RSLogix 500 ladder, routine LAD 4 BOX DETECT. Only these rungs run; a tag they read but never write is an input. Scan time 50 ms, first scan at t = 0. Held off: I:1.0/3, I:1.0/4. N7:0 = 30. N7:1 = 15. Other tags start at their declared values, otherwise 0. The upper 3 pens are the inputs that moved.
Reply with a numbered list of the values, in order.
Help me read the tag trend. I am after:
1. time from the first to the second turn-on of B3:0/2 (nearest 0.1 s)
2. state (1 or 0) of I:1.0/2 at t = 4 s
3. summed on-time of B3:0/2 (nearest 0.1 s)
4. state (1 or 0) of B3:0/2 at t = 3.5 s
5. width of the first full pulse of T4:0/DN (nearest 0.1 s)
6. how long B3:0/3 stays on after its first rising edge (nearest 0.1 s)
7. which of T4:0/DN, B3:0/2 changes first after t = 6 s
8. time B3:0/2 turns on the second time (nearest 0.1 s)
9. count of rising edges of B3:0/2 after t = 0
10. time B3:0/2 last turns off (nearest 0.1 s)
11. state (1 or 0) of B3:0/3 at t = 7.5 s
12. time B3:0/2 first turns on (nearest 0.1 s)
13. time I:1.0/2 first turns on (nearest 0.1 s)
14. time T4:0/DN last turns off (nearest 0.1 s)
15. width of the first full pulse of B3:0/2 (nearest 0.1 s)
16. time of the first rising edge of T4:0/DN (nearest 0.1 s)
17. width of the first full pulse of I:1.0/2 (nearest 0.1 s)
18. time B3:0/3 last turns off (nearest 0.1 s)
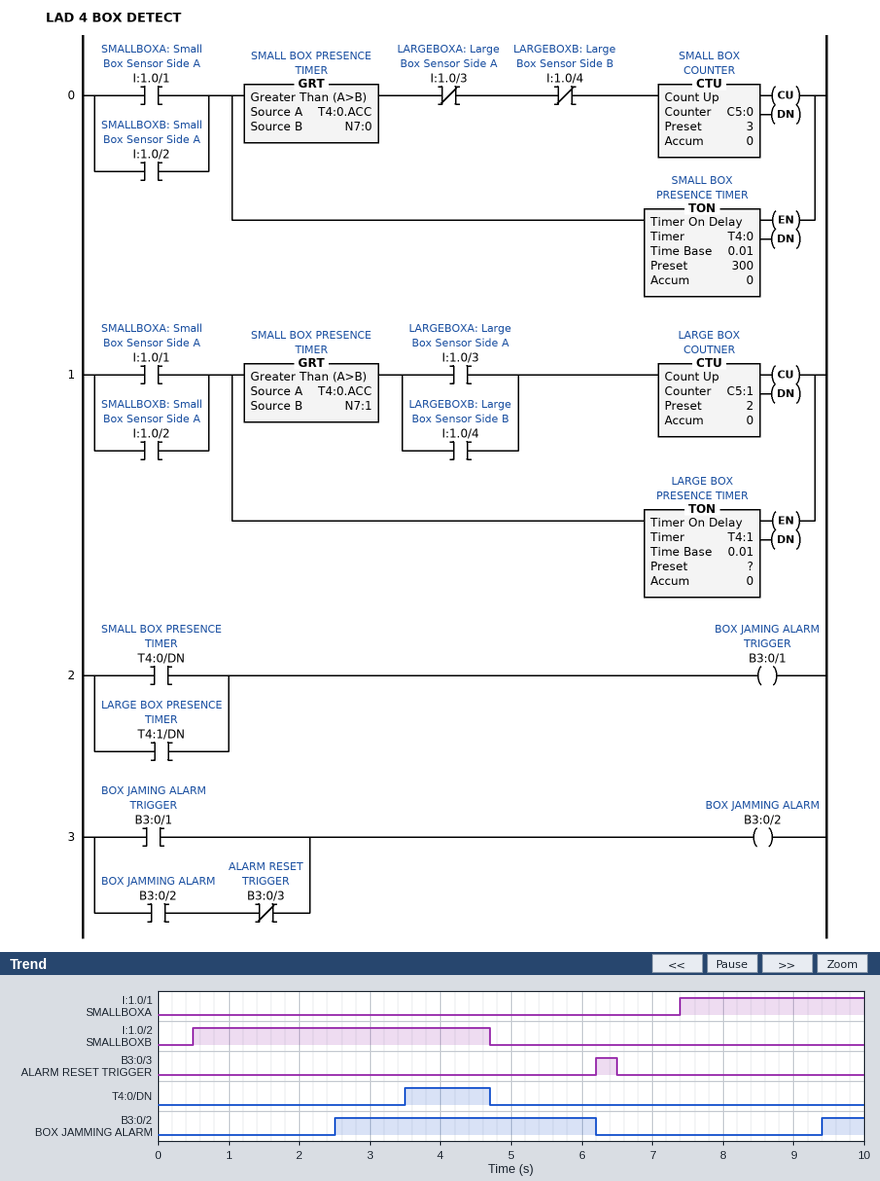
1. 6.9 s
2. 1
3. 4.3 s
4. 1
5. 1.2 s
6. 0.3 s
7. B3:0/2
8. 9.4 s
9. 2
10. 6.2 s
11. 0
12. 2.5 s
13. 0.5 s
14. 4.7 s
15. 3.7 s
16. 3.5 s
17. 4.2 s
18. 6.5 s
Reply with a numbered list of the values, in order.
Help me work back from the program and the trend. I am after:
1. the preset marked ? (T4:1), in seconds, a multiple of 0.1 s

1. 2.0 s
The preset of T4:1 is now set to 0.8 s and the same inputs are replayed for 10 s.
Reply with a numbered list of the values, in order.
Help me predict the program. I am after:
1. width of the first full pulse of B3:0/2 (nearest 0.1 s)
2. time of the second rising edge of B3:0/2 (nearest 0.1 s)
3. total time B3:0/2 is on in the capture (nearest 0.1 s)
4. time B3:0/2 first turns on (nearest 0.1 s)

1. 4.9 s
2. 8.2 s
3. 6.7 s
4. 1.3 s
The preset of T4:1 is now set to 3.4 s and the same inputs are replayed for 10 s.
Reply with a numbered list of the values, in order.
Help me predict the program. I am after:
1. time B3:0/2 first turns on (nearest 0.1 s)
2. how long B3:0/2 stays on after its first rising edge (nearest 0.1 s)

1. 3.5 s
2. 2.7 s
